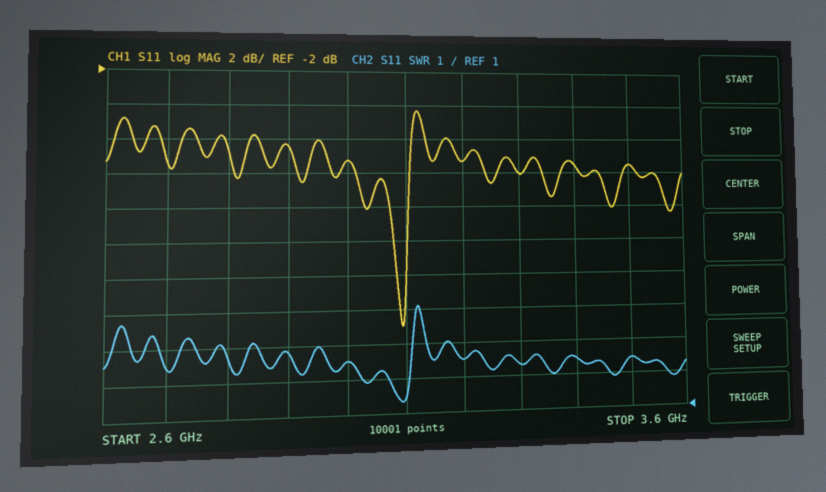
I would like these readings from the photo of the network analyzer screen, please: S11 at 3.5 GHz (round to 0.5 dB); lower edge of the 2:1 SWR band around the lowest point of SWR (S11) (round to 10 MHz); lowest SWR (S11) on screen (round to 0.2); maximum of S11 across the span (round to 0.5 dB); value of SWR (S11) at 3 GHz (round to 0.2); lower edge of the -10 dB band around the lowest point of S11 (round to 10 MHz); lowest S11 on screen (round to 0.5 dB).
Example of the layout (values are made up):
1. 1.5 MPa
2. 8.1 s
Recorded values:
1. -7.5 dB
2. 3.07 GHz
3. 1.4
4. -4.5 dB
5. 2.6
6. 3.07 GHz
7. -17.0 dB
